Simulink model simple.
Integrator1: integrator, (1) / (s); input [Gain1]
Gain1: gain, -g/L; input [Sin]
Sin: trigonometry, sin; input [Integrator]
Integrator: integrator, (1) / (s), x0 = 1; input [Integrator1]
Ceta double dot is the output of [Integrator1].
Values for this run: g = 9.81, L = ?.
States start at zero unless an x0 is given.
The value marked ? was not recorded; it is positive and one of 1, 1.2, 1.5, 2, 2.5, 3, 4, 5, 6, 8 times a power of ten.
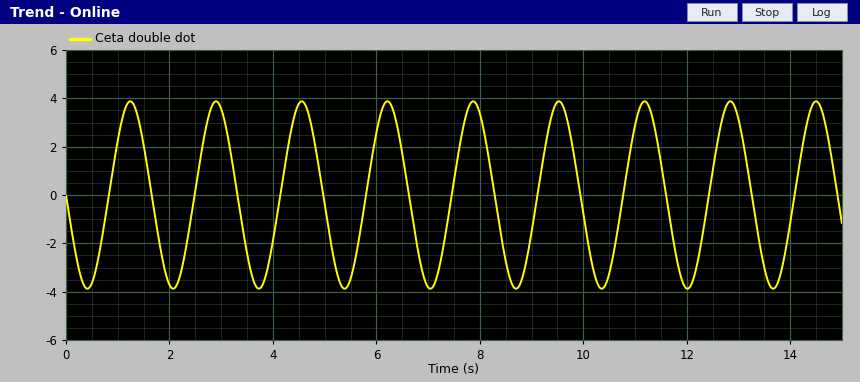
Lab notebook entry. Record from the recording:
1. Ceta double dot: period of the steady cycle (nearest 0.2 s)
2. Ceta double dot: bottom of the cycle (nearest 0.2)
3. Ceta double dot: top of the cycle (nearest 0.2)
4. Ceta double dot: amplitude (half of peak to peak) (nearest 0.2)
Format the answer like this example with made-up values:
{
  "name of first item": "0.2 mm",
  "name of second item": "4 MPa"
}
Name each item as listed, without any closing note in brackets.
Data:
{
  "Ceta double dot: period of the steady cycle": "1.6 s",
  "Ceta double dot: bottom of the cycle": "-3.8",
  "Ceta double dot: top of the cycle": "3.8",
  "Ceta double dot: amplitude (half of peak to peak)": "3.8"
}
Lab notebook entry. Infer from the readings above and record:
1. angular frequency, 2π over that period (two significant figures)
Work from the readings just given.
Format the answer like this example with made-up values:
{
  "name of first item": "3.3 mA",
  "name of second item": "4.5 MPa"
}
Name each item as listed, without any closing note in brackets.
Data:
{
  "angular frequency, 2π over that period": "3.9 rad/s"
}
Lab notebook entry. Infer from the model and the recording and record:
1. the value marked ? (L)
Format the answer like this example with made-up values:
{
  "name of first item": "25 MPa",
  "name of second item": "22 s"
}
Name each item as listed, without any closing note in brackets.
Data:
{
  "the value marked ?": "0.6"
}
